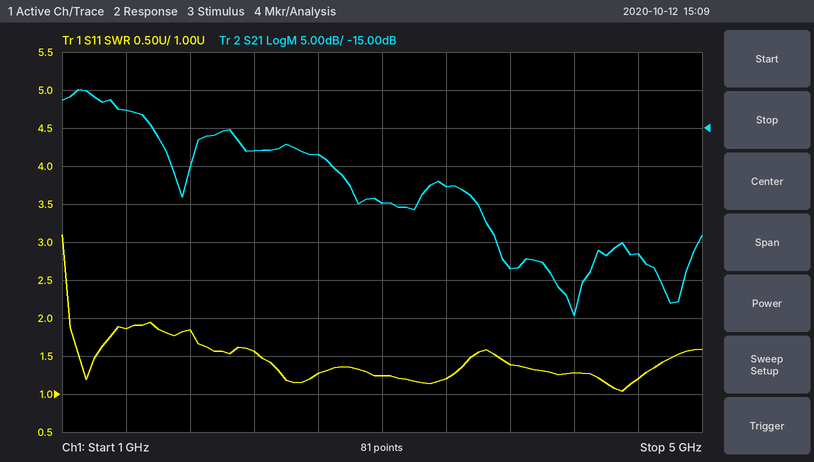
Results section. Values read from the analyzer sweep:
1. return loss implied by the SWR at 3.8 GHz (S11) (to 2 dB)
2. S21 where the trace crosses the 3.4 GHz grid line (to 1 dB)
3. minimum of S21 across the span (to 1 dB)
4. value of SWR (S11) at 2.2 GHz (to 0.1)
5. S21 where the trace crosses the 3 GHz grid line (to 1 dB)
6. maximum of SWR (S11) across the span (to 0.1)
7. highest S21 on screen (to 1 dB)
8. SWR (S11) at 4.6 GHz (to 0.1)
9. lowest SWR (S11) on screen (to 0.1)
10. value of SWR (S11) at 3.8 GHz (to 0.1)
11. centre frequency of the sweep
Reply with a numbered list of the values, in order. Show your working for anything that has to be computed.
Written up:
1. −20 log10((1.4 − 1)/(1.4 + 1)) ≈ 16 dB
2. -23 dB
3. -40 dB
4. 1.6
5. -25 dB
6. 3.1
7. -10 dB
8. 1.2
9. 1.0
10. 1.4
11. 3 GHz
